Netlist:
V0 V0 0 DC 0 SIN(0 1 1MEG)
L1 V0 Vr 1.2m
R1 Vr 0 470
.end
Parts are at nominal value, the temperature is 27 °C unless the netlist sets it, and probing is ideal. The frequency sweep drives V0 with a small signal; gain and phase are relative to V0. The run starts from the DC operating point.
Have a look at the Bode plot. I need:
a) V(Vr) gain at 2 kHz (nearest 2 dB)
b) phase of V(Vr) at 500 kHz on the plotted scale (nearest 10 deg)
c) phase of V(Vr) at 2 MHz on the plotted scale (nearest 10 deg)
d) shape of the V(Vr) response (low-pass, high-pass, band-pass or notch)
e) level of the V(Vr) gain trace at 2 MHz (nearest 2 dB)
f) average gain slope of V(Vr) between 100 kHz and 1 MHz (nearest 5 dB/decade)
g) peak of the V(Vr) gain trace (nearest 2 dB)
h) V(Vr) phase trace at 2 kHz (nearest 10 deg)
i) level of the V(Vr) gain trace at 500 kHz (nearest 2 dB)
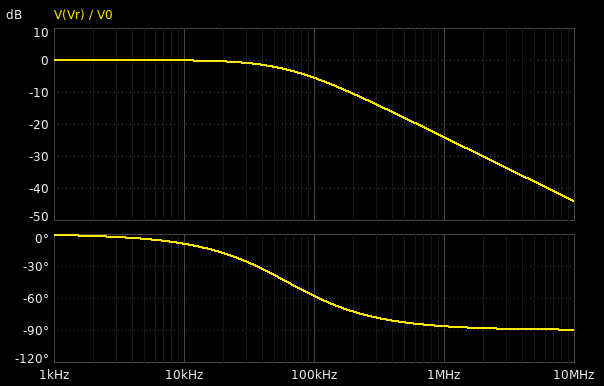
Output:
0 dB
-80 deg
-90 deg
low-pass
-30 dB
-20 dB/decade
0 dB
0 deg
-18 dB
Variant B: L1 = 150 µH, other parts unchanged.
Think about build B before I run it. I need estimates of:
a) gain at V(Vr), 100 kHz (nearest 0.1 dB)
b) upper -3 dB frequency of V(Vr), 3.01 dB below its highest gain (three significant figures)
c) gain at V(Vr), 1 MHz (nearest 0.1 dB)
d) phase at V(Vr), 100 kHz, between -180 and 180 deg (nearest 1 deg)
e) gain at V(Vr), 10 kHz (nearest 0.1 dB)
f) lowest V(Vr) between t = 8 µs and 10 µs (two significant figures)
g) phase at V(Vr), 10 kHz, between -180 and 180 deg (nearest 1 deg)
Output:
-0.2 dB
499 kHz
-7.0 dB
-11 deg
0 dB
-450 mV
-1 deg
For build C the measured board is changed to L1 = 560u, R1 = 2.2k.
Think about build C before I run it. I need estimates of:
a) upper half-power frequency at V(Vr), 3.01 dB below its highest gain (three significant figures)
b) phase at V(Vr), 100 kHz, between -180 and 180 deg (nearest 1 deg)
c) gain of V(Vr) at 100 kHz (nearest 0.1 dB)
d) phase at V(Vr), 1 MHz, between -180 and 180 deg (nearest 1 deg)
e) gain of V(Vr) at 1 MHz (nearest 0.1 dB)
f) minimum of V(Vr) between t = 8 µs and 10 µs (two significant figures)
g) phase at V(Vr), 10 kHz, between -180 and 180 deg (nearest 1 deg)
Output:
625 kHz
-9 deg
-0.1 dB
-58 deg
-5.5 dB
-530 mV
-1 deg
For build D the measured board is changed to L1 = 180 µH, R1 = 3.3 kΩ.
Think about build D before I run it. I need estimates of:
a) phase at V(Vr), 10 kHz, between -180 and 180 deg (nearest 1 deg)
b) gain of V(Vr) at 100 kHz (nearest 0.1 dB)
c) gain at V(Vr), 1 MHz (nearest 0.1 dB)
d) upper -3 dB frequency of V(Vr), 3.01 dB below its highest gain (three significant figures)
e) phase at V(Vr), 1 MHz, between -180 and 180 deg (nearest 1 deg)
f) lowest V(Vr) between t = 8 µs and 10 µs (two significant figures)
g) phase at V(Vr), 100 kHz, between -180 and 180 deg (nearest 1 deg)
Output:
0 deg
0 dB
-0.5 dB
2.92 MHz
-19 deg
-950 mV
-2 deg
